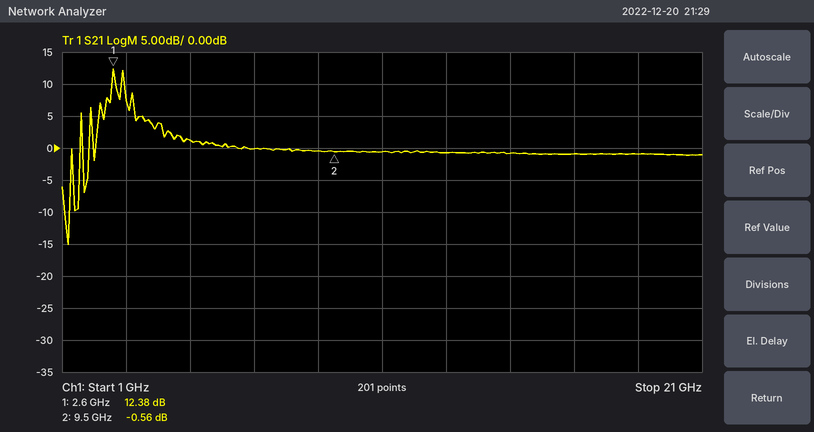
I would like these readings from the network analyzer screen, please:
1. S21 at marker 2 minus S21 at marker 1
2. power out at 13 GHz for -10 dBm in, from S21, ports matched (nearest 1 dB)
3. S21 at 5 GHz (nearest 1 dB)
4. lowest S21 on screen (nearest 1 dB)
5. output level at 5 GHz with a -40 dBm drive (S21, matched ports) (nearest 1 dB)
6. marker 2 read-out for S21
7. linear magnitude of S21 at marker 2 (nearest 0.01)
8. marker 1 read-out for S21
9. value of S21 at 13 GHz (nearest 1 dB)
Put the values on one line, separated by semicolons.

-12.94 dB; -11 dBm; 1 dB; -15 dB; -39 dBm; -0.56 dB; 0.94; 12.38 dB; -1 dB
